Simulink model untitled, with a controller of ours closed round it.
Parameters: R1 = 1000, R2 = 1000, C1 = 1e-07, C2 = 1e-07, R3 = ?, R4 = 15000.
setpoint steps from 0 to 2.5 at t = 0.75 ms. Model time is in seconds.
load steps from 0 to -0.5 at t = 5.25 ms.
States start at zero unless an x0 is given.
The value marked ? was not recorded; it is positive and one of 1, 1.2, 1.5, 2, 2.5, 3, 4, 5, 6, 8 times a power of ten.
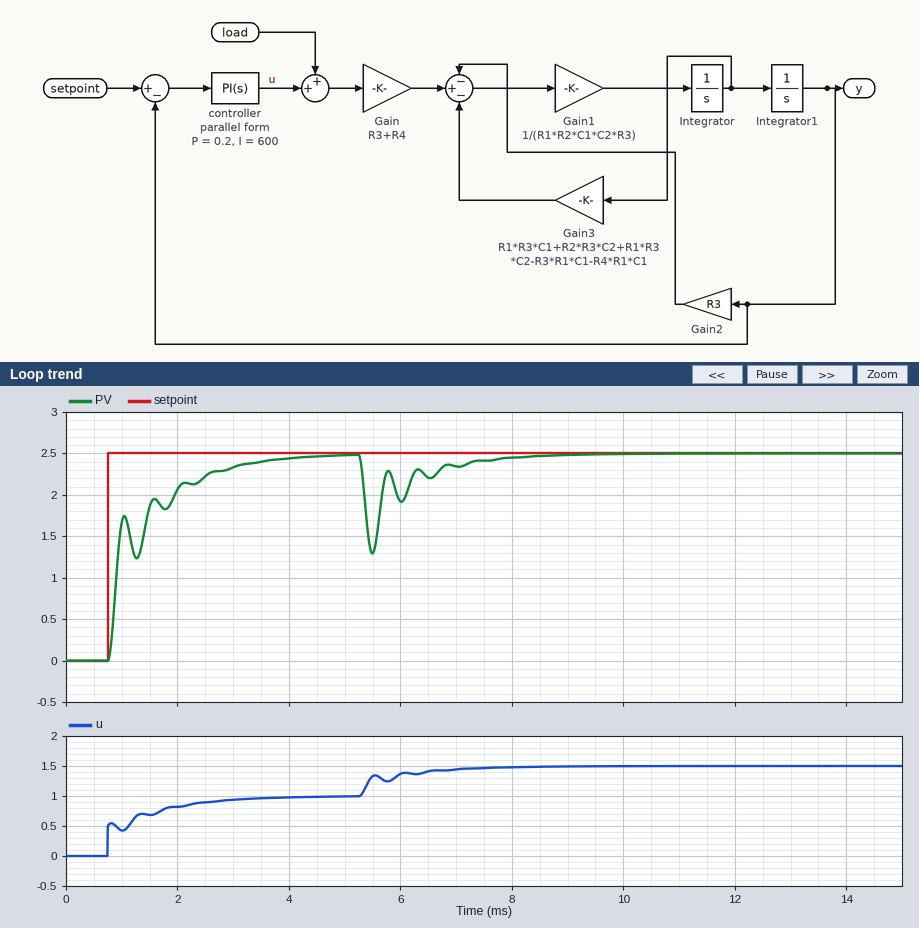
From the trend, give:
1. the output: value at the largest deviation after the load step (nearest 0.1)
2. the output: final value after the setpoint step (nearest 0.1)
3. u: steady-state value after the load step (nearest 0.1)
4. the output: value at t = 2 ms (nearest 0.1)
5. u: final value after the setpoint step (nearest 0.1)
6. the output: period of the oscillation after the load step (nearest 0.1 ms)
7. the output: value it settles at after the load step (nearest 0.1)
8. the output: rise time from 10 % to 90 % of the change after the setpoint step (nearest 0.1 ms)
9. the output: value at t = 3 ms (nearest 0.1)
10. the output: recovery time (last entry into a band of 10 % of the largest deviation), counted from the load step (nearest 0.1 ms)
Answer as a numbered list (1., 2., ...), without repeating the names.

1. 1.3
2. 2.5
3. 1.5
4. 2.1
5. 1.0
6. 0.5 ms
7. 2.5
8. 1.7 ms
9. 2.3
10. 2.0 ms
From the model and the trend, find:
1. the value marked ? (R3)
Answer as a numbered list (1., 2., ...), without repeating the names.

1. 10000
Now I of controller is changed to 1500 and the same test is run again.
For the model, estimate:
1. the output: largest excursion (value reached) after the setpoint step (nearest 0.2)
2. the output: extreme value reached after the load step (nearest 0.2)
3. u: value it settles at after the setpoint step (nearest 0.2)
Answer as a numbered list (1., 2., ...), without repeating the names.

1. 2.6
2. 1.4
3. 1.0
